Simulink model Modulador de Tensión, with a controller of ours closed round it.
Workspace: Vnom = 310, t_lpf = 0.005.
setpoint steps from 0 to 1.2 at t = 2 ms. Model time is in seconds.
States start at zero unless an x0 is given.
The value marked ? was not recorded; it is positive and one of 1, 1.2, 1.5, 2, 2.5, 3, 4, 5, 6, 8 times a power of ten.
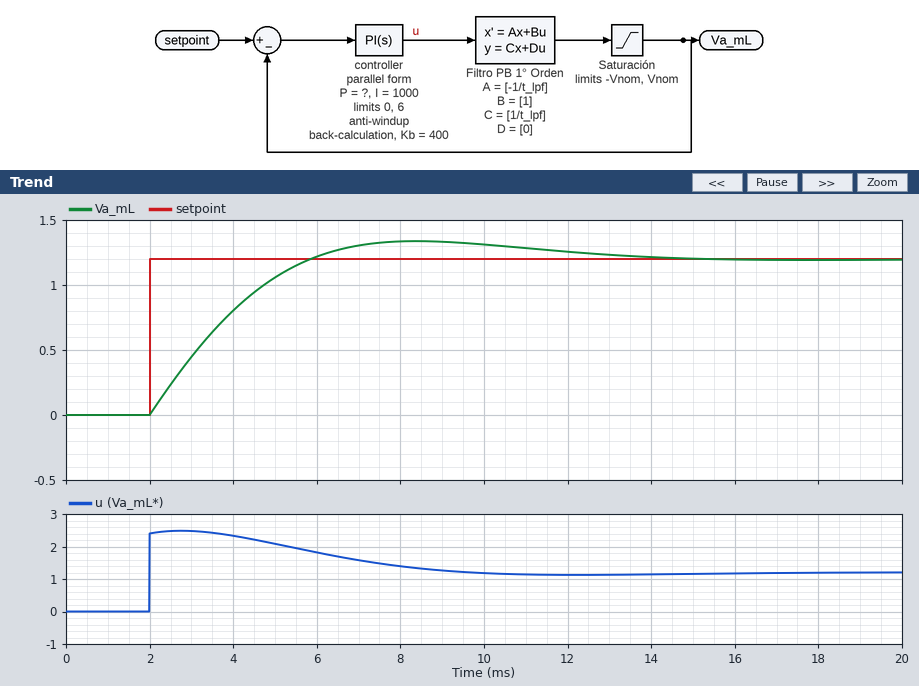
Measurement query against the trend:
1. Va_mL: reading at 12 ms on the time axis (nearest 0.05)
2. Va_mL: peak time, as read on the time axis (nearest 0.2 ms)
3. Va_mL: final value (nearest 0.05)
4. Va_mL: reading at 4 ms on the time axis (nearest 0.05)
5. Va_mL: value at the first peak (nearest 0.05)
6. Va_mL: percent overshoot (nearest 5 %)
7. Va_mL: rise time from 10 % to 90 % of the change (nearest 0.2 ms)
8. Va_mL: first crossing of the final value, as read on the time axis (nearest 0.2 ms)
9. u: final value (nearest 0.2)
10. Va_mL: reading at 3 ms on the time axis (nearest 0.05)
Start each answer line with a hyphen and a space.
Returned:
- 1.25
- 8.4 ms
- 1.20
- 0.80
- 1.35
- 10 %
- 2.8 ms
- 5.8 ms
- 1.2
- 0.45
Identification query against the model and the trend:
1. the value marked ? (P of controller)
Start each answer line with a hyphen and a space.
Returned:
- 2
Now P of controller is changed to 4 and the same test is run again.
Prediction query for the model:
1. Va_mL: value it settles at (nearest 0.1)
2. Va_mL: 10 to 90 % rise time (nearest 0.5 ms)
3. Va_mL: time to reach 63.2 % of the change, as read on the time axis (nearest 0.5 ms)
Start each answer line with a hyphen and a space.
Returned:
- 1.2
- 2.5 ms
- 3.0 ms
